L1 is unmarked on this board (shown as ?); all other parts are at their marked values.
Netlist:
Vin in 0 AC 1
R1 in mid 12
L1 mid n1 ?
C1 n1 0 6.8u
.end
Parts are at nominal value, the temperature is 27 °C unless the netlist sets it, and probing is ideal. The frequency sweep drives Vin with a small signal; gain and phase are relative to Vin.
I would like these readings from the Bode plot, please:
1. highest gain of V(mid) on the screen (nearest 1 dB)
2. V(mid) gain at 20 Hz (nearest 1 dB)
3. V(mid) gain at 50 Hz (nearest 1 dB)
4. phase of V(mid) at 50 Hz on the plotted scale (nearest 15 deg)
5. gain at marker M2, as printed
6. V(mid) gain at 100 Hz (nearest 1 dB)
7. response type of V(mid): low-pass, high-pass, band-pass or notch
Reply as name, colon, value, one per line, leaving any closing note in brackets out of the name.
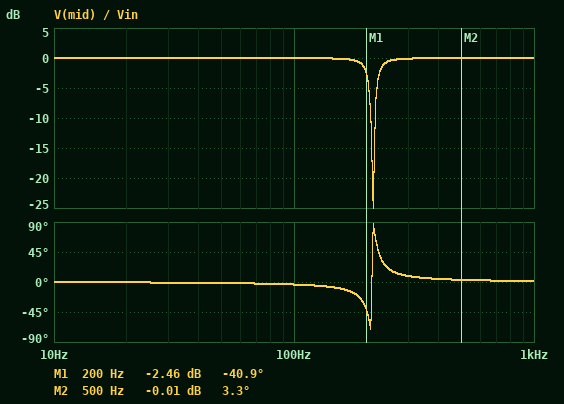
highest gain of V(mid) on the screen: 0 dB
V(mid) gain at 20 Hz: 0 dB
V(mid) gain at 50 Hz: 0 dB
phase of V(mid) at 50 Hz on the plotted scale: 0 deg
gain at marker M2, as printed: -0.01 dB
V(mid) gain at 100 Hz: 0 dB
response type of V(mid): low-pass, high-pass, band-pass or notch: notch
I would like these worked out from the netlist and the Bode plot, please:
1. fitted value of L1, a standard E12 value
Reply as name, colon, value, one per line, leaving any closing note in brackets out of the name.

fitted value of L1, a standard E12 value: 82 mH
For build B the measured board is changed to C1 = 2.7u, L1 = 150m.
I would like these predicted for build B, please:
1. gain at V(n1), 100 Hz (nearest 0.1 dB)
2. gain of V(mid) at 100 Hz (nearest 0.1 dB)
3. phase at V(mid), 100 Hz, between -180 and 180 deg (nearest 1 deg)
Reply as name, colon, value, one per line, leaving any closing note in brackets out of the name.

gain at V(n1), 100 Hz: 1.5 dB
gain of V(mid) at 100 Hz: 0 dB
phase at V(mid), 100 Hz, between -180 and 180 deg: -1 deg
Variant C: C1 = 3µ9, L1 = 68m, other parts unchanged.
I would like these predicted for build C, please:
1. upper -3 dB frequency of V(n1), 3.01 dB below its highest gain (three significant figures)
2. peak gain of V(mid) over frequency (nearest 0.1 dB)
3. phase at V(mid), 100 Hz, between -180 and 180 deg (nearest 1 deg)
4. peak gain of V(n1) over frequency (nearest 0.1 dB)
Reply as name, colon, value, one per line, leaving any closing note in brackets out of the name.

upper -3 dB frequency of V(n1), 3.01 dB below its highest gain: 322 Hz
peak gain of V(mid) over frequency: 0 dB
phase at V(mid), 100 Hz, between -180 and 180 deg: -2 deg
peak gain of V(n1) over frequency: 20.8 dB
